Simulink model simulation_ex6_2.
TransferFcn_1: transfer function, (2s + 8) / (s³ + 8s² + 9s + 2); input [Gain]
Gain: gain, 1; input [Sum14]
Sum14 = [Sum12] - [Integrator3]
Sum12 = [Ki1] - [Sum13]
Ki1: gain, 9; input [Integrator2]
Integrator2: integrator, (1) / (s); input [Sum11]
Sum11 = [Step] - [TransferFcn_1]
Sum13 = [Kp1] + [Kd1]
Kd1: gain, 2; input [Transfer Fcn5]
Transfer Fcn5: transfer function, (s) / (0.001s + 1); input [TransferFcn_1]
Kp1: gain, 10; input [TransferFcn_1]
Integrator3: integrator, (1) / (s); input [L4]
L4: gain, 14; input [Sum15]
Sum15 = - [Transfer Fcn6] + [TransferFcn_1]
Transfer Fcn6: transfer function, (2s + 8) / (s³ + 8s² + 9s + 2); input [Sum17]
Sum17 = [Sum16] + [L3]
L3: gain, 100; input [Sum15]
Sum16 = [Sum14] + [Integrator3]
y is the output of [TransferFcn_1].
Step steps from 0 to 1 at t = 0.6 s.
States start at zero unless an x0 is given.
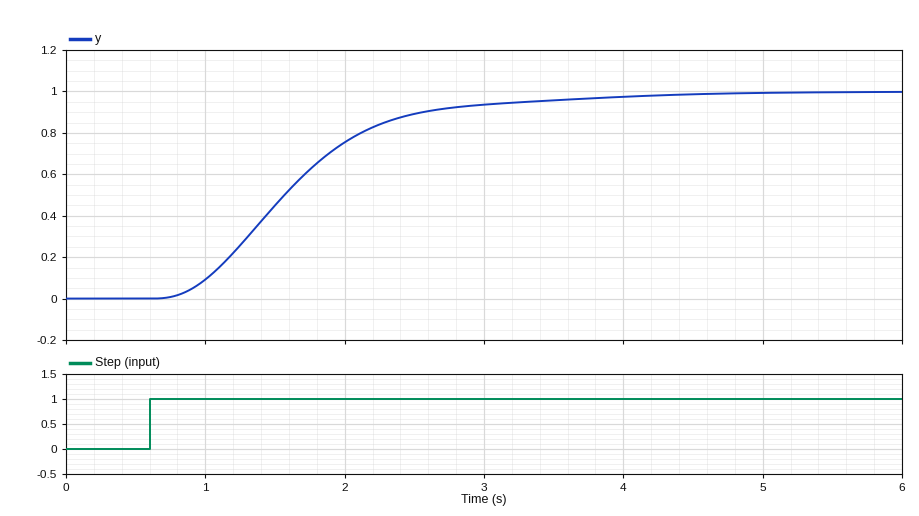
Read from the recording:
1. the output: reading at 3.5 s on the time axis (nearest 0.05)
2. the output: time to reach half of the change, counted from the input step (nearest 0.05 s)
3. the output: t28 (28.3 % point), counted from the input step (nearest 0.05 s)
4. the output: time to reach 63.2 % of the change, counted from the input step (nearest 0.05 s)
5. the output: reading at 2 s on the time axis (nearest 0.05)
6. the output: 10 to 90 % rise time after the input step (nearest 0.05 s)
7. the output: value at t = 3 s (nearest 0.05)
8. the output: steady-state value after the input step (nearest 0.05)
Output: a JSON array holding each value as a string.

["0.95", "0.95 s", "0.70 s", "1.15 s", "0.75", "1.55 s", "0.95", "1.00"]
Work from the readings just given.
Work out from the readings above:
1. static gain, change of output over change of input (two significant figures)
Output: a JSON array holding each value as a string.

["1.0"]
